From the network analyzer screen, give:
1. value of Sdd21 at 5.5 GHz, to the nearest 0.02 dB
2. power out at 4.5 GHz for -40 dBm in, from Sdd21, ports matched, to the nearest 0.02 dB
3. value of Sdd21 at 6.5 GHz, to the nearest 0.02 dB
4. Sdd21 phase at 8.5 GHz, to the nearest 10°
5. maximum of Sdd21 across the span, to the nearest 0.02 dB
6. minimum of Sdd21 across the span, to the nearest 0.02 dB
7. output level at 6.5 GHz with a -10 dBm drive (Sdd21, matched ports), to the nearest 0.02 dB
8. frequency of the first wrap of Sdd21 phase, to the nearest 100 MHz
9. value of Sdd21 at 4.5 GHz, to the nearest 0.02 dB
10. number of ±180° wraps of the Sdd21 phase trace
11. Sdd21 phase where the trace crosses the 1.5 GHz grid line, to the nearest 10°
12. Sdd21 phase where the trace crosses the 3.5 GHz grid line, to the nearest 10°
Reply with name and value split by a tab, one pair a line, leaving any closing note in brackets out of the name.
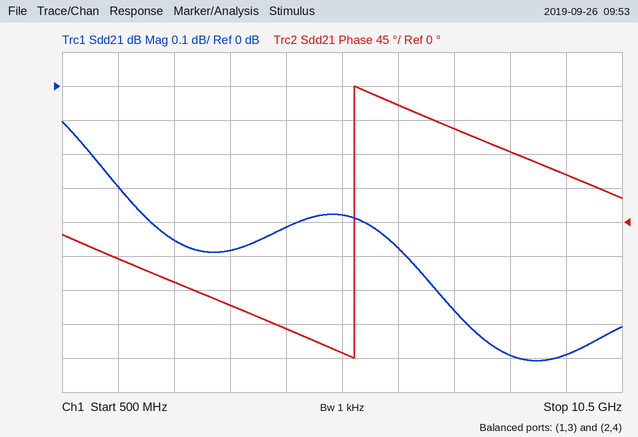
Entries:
value of Sdd21 at 5.5 GHz, to the nearest 0.02 dB	-0.38 dB
power out at 4.5 GHz for -40 dBm in, from Sdd21, ports matched, to the nearest 0.02 dB	-40.42 dBm
value of Sdd21 at 6.5 GHz, to the nearest 0.02 dB	-0.48 dB
Sdd21 phase at 8.5 GHz, to the nearest 10°	90°
maximum of Sdd21 across the span, to the nearest 0.02 dB	-0.10 dB
minimum of Sdd21 across the span, to the nearest 0.02 dB	-0.80 dB
output level at 6.5 GHz with a -10 dBm drive (Sdd21, matched ports), to the nearest 0.02 dB	-10.48 dBm
frequency of the first wrap of Sdd21 phase, to the nearest 100 MHz	5.7 GHz
value of Sdd21 at 4.5 GHz, to the nearest 0.02 dB	-0.42 dB
number of ±180° wraps of the Sdd21 phase trace	1
Sdd21 phase where the trace crosses the 1.5 GHz grid line, to the nearest 10°	-50°
Sdd21 phase where the trace crosses the 3.5 GHz grid line, to the nearest 10°	-110°
